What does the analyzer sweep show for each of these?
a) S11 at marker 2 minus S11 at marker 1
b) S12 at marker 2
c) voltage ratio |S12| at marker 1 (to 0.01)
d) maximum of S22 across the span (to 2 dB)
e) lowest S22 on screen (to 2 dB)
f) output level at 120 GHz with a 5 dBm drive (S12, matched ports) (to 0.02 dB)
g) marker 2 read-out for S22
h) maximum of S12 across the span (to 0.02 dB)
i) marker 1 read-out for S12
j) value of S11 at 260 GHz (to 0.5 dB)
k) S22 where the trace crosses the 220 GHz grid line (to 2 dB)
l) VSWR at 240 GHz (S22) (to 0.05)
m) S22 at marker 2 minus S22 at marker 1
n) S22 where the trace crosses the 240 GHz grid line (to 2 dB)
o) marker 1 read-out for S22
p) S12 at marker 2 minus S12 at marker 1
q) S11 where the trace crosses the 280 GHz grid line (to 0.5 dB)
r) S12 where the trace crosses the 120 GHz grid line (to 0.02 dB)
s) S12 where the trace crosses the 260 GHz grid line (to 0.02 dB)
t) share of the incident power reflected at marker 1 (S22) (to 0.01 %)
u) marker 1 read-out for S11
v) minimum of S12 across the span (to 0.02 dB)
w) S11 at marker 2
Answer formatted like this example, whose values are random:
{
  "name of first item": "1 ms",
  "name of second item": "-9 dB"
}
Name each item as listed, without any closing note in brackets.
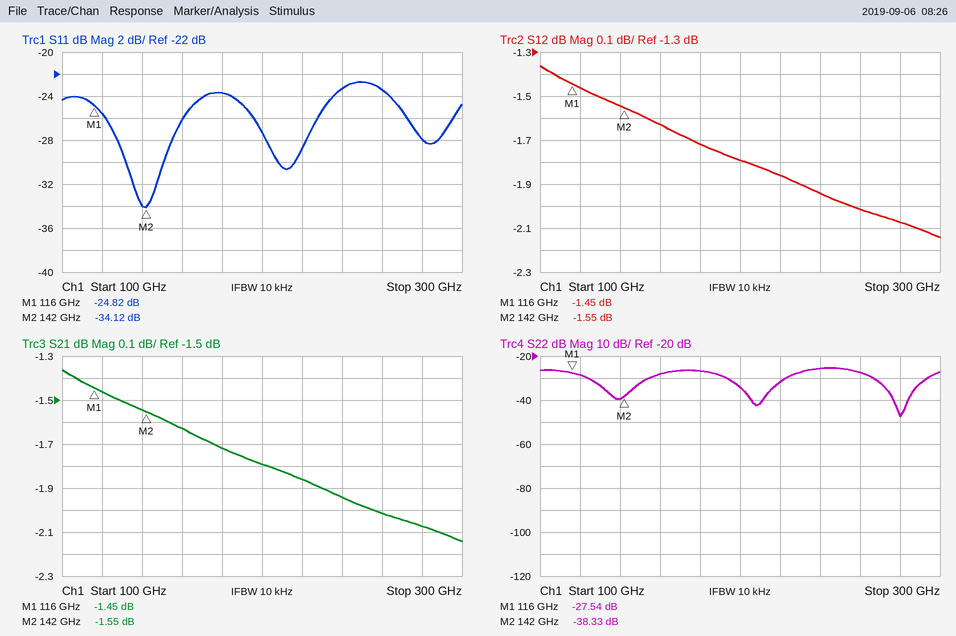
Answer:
{
  "S11 at marker 2 minus S11 at marker 1": "-9.30 dB",
  "S12 at marker 2": "-1.55 dB",
  "voltage ratio |S12| at marker 1": "0.85",
  "maximum of S22 across the span": "-26 dB",
  "lowest S22 on screen": "-48 dB",
  "output level at 120 GHz with a 5 dBm drive (S12, matched ports)": "3.54 dBm",
  "marker 2 read-out for S22": "-38.33 dB",
  "maximum of S12 across the span": "-1.36 dB",
  "marker 1 read-out for S12": "-1.45 dB",
  "value of S11 at 260 GHz": "-23.5 dB",
  "S22 where the trace crosses the 220 GHz grid line": "-32 dB",
  "VSWR at 240 GHz (S22)": "1.10",
  "S22 at marker 2 minus S22 at marker 1": "-10.79 dB",
  "S22 where the trace crosses the 240 GHz grid line": "-26 dB",
  "marker 1 read-out for S22": "-27.54 dB",
  "S12 at marker 2 minus S12 at marker 1": "-0.10 dB",
  "S11 where the trace crosses the 280 GHz grid line": "-28.0 dB",
  "S12 where the trace crosses the 120 GHz grid line": "-1.46 dB",
  "S12 where the trace crosses the 260 GHz grid line": "-2.02 dB",
  "share of the incident power reflected at marker 1 (S22)": "0.18 %",
  "marker 1 read-out for S11": "-24.82 dB",
  "minimum of S12 across the span": "-2.14 dB",
  "S11 at marker 2": "-34.12 dB"
}
